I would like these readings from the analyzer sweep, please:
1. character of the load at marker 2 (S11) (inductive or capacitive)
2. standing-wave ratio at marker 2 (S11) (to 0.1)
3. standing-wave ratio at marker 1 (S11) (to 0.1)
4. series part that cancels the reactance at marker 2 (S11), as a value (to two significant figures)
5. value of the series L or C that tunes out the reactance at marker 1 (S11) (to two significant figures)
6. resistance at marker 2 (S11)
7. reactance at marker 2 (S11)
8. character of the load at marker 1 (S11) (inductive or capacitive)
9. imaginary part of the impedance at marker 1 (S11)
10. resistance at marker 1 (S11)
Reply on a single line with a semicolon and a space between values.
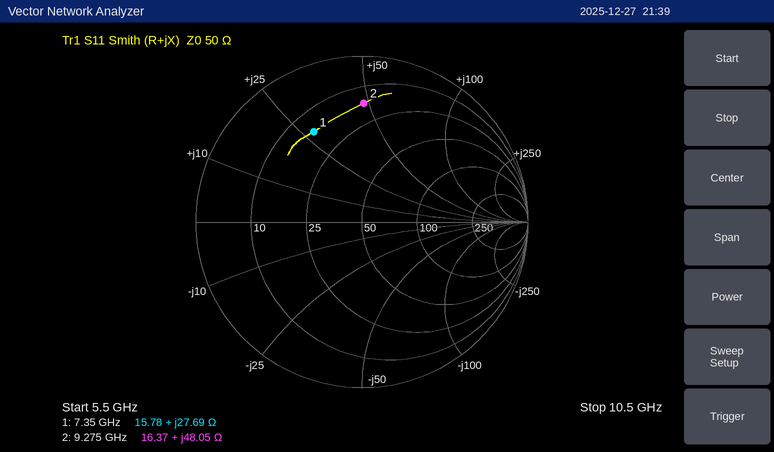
inductive; 6.0; 4.2; 360 fF; 780 fF; 16.37 Ω; +48.05 Ω; inductive; +27.69 Ω; 15.78 Ω
